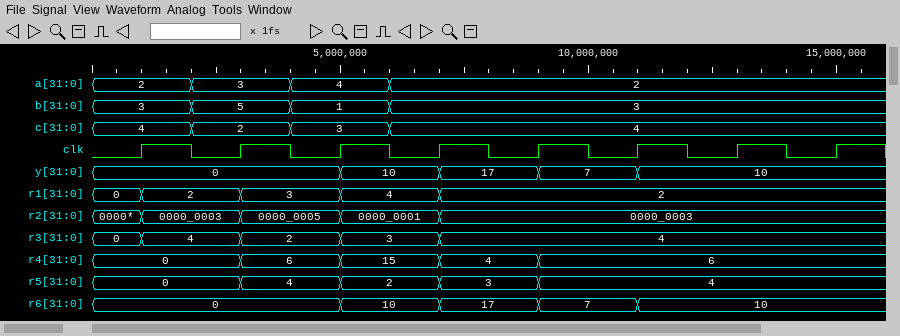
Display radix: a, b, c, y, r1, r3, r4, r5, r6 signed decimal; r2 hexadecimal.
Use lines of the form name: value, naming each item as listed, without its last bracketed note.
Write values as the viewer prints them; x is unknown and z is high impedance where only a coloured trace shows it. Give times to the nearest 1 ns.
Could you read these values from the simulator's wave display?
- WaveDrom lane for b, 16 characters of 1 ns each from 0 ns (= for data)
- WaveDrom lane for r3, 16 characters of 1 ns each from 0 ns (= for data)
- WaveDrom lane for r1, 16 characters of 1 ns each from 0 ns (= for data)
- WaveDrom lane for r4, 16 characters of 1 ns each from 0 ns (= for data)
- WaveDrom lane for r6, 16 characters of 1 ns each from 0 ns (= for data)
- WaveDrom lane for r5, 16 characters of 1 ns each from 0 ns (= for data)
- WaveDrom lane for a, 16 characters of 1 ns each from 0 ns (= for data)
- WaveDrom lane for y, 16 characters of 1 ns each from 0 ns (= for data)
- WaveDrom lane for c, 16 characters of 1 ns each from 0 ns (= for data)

WaveDrom lane for b, 16 characters of 1 ns each from 0 ns: {name: 'b', wave: '=.=.=.=.........', data: '3 5 1 3'}
WaveDrom lane for r3, 16 characters of 1 ns each from 0 ns: {name: 'r3', wave: '==.=.=.=........', data: '0 4 2 3 4'}
WaveDrom lane for r1, 16 characters of 1 ns each from 0 ns: {name: 'r1', wave: '==.=.=.=........', data: '0 2 3 4 2'}
WaveDrom lane for r4, 16 characters of 1 ns each from 0 ns: {name: 'r4', wave: '=..=.=.=.=......', data: '0 6 15 4 6'}
WaveDrom lane for r6, 16 characters of 1 ns each from 0 ns: {name: 'r6', wave: '=....=.=.=.=....', data: '0 10 17 7 10'}
WaveDrom lane for r5, 16 characters of 1 ns each from 0 ns: {name: 'r5', wave: '=..=.=.=.=......', data: '0 4 2 3 4'}
WaveDrom lane for a, 16 characters of 1 ns each from 0 ns: {name: 'a', wave: '=.=.=.=.........', data: '2 3 4 2'}
WaveDrom lane for y, 16 characters of 1 ns each from 0 ns: {name: 'y', wave: '=....=.=.=.=....', data: '0 10 17 7 10'}
WaveDrom lane for c, 16 characters of 1 ns each from 0 ns: {name: 'c', wave: '=.=.=.=.........', data: '4 2 3 4'}
